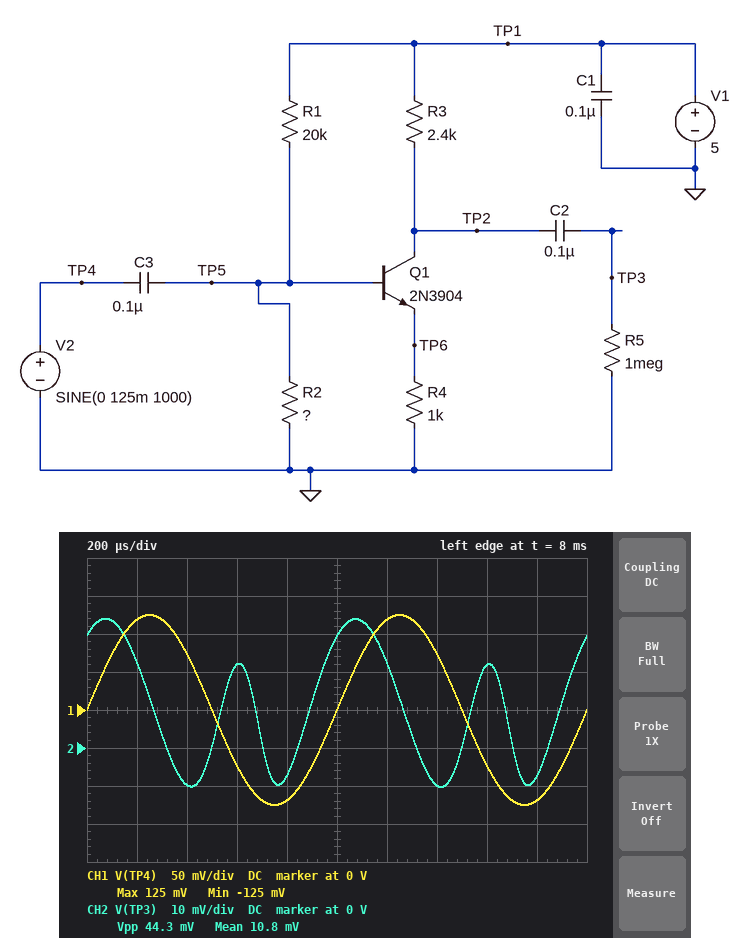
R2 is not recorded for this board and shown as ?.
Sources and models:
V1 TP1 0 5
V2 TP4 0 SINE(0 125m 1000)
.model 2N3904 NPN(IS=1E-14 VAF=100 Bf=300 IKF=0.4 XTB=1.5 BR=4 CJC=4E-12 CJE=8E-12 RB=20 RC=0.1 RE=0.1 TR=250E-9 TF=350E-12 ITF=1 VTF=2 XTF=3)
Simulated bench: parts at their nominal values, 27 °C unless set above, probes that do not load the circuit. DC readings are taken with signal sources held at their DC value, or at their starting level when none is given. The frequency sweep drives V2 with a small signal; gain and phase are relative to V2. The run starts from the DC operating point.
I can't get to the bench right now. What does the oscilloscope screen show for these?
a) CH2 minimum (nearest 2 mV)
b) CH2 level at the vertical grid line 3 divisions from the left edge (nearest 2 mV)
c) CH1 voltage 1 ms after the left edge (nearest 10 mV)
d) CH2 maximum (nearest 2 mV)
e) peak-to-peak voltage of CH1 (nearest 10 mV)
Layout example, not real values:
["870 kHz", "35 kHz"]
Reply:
["-10 mV", "22 mV", "0 V", "34 mV", "250 mV"]
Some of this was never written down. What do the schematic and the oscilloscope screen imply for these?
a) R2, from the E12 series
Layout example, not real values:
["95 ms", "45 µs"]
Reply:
["27 kΩ"]
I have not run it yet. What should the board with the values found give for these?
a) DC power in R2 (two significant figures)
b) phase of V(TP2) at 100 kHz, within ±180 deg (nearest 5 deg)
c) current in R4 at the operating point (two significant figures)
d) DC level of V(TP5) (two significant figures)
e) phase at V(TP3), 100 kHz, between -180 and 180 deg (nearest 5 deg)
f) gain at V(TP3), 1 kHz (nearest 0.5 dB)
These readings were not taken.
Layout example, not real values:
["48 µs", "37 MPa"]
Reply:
["170 µW", "20 deg", "1.5 mA", "2.2 V", "20 deg", "-13.0 dB"]
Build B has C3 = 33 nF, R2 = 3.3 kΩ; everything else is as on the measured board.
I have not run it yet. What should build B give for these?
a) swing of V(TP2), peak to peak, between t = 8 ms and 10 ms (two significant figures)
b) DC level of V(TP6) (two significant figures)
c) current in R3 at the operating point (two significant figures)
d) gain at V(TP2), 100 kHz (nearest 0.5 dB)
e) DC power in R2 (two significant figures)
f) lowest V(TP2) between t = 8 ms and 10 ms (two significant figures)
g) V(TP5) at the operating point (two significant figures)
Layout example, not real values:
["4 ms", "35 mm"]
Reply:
["240 mV", "110 mV", "110 µA", "5.5 dB", "150 µW", "4.6 V", "710 mV"]
